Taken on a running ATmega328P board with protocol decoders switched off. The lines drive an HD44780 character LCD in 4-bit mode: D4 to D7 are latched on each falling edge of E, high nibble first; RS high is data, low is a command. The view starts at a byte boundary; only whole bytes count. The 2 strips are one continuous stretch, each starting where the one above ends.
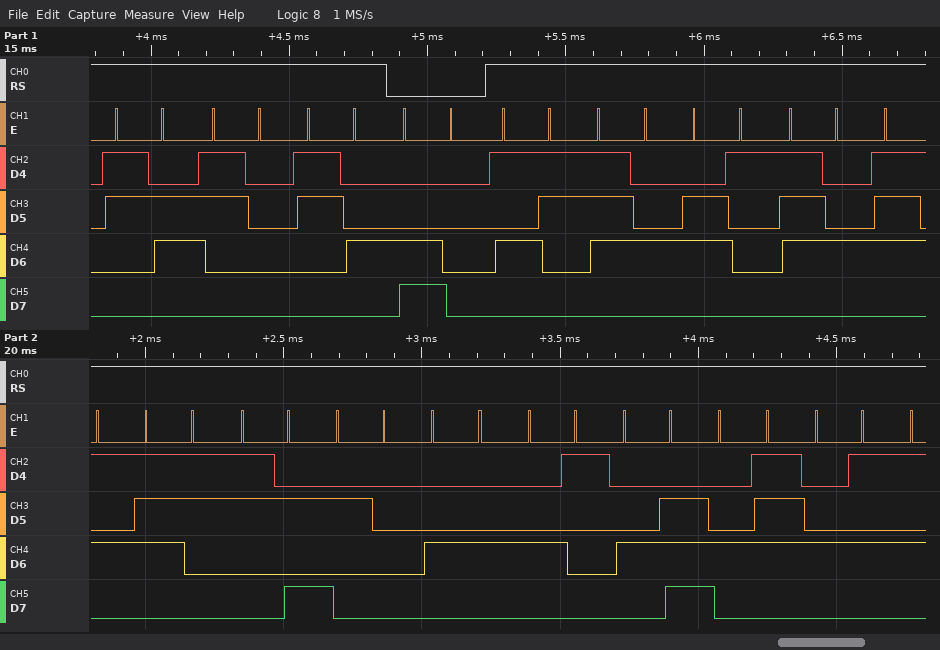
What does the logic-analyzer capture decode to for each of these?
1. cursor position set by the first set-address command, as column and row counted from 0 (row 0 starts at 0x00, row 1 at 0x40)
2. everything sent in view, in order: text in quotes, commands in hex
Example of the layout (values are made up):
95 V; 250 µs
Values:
column 0, row 1; "604" 0xC0 "Status: DANGE"
